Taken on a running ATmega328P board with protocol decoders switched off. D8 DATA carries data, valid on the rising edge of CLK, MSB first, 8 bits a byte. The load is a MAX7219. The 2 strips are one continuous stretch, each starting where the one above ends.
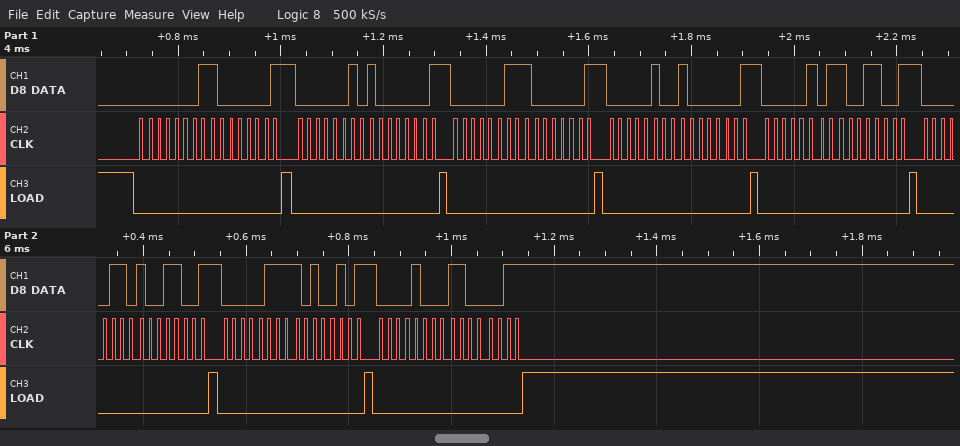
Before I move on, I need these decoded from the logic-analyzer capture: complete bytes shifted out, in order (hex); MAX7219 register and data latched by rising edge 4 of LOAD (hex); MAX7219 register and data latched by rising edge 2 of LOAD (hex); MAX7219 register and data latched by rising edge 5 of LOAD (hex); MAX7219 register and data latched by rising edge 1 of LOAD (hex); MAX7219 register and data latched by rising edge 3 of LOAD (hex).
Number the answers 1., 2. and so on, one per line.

1. 01 81 02 81 03 81 04 81 05 99 06 99 07 A5 08 C3
2. register 0x4, data 0x81
3. register 0x2, data 0x81
4. register 0x5, data 0x99
5. register 0x1, data 0x81
6. register 0x3, data 0x81
